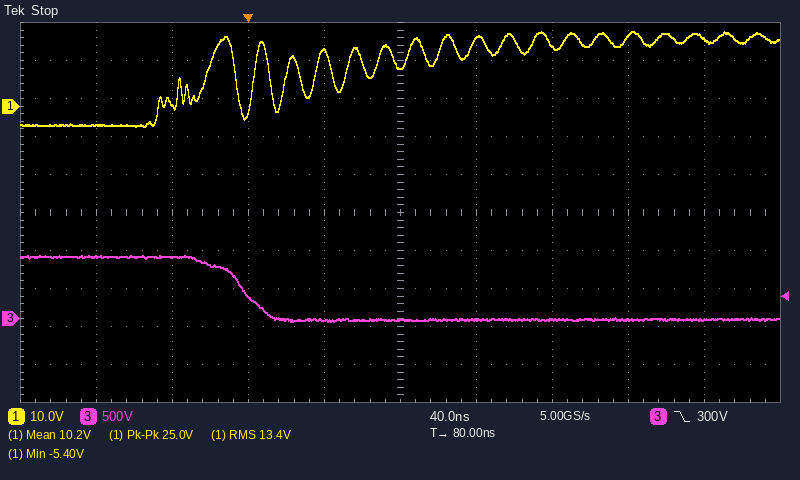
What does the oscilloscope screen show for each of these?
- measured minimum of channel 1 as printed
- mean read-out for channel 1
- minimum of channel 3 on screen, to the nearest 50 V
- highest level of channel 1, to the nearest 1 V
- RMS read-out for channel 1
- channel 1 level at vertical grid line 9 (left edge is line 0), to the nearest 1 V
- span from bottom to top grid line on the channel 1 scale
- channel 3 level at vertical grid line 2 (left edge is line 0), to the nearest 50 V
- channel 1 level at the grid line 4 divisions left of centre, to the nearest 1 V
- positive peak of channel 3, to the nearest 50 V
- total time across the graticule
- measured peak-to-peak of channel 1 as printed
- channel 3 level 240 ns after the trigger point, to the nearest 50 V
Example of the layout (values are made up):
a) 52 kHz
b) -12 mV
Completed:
a) -5.40 V
b) 10.2 V
c) -50 V
d) 20 V
e) 13.4 V
f) 18 V
g) 100 V
h) 800 V
i) -5 V
j) 850 V
k) 400 ns
l) 25.0 V
m) 0 V
